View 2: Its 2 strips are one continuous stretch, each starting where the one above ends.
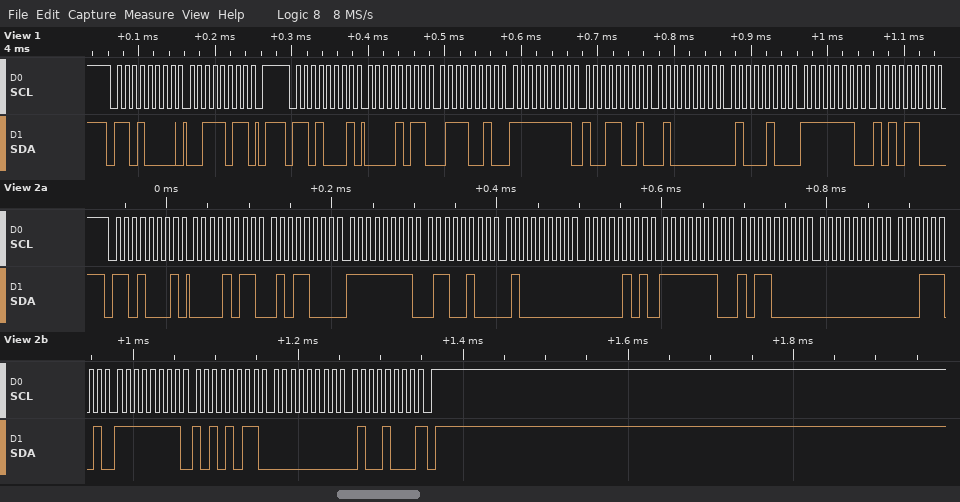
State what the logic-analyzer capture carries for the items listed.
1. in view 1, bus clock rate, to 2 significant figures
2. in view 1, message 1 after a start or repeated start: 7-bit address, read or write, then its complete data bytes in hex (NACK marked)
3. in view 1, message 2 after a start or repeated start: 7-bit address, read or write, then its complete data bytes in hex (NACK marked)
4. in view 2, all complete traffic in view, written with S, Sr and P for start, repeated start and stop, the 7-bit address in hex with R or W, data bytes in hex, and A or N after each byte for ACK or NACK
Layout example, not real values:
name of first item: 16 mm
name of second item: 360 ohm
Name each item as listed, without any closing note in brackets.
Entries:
in view 1, bus clock rate, to 2 significant figures: 100 kHz
in view 1, message 1 after a start or repeated start: 7-bit address, read or write, then its complete data bytes in hex: 0x68 write: 3B
in view 1, message 2 after a start or repeated start: 7-bit address, read or write, then its complete data bytes in hex: 0x68 read: 0B 72 FF 99 40 44 FE AC
in view 2, all complete traffic in view, written with S, Sr and P for start, repeated start and stop, the 7-bit address in hex with R or W, data bytes in hex, and A or N after each byte for ACK or NACK: S 68R A 0B A 58 A FF A 64 A 40 A 05 A FE A B0 A 00 A 1D A FF A AB A 00 A 48 N P
